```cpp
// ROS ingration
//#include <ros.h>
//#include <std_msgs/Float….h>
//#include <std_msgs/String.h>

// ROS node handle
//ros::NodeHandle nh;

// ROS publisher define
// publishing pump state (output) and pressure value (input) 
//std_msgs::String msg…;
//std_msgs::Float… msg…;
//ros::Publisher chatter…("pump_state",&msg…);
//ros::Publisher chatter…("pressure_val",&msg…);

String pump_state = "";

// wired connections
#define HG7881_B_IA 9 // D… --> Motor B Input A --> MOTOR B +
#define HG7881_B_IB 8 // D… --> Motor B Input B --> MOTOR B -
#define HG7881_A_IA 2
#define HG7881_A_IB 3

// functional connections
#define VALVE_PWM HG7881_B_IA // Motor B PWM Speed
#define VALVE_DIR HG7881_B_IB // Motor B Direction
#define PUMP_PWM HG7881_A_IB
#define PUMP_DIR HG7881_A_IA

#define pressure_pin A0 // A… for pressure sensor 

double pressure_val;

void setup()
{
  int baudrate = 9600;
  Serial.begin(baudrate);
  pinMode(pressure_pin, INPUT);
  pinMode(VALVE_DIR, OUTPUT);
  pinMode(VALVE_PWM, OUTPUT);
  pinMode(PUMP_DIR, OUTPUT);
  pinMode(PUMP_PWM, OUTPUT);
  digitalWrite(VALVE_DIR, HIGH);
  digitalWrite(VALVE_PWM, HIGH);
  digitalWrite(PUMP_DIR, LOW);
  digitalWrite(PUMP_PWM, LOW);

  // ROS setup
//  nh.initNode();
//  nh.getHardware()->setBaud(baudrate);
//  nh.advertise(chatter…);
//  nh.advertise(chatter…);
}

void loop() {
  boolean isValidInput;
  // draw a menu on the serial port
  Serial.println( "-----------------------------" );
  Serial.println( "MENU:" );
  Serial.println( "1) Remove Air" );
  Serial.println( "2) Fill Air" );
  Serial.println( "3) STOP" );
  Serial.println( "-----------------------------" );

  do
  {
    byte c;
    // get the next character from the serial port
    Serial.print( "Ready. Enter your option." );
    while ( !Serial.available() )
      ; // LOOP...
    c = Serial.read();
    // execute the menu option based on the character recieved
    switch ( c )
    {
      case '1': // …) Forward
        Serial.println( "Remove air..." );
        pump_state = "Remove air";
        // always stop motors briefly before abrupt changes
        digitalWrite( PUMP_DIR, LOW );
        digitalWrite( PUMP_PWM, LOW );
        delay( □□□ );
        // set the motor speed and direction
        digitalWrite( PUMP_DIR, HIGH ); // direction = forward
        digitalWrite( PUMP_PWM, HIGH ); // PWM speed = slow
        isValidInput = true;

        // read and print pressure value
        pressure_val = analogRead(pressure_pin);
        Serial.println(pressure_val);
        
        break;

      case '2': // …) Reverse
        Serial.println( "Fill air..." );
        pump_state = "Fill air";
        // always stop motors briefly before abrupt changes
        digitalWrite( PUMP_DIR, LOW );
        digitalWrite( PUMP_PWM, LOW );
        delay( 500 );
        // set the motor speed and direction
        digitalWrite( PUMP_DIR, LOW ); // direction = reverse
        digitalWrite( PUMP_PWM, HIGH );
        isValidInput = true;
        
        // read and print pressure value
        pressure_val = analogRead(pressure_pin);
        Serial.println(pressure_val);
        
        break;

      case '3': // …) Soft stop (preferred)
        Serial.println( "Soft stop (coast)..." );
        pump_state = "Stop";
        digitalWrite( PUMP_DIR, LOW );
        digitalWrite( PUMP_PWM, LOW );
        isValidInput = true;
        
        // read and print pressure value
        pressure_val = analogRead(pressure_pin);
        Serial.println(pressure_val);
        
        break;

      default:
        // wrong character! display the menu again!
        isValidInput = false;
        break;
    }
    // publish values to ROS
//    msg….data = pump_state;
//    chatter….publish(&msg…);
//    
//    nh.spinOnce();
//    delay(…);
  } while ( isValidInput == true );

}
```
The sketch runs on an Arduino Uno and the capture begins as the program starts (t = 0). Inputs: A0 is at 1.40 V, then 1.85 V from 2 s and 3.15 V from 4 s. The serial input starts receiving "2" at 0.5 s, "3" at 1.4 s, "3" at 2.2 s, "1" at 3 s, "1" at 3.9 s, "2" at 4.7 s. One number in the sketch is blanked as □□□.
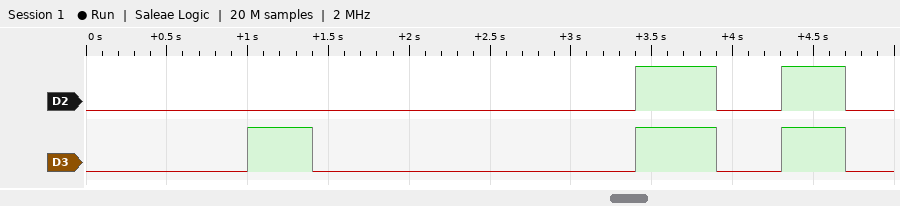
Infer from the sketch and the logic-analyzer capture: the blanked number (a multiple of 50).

400
